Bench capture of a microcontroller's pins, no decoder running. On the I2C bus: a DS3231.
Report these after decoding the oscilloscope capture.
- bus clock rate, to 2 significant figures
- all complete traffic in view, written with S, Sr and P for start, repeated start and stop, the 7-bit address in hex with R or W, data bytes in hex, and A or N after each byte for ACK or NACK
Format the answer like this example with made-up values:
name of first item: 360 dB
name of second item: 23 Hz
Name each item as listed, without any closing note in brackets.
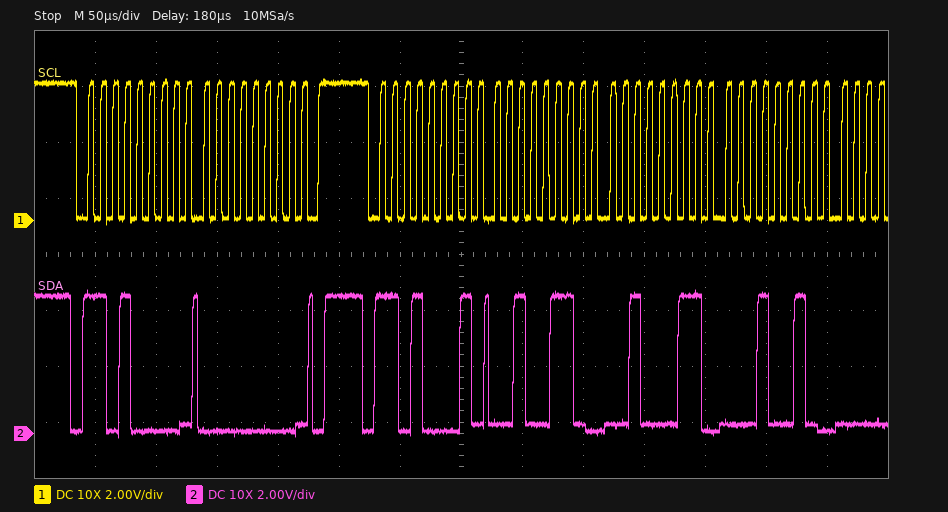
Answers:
bus clock rate, to 2 significant figures: 100 kHz
all complete traffic in view, written with S, Sr and P for start, repeated start and stop, the 7-bit address in hex with R or W, data bytes in hex, and A or N after each byte for ACK or NACK: S 68W A 00 A P S 68R A 26 A 23 A 12 A
